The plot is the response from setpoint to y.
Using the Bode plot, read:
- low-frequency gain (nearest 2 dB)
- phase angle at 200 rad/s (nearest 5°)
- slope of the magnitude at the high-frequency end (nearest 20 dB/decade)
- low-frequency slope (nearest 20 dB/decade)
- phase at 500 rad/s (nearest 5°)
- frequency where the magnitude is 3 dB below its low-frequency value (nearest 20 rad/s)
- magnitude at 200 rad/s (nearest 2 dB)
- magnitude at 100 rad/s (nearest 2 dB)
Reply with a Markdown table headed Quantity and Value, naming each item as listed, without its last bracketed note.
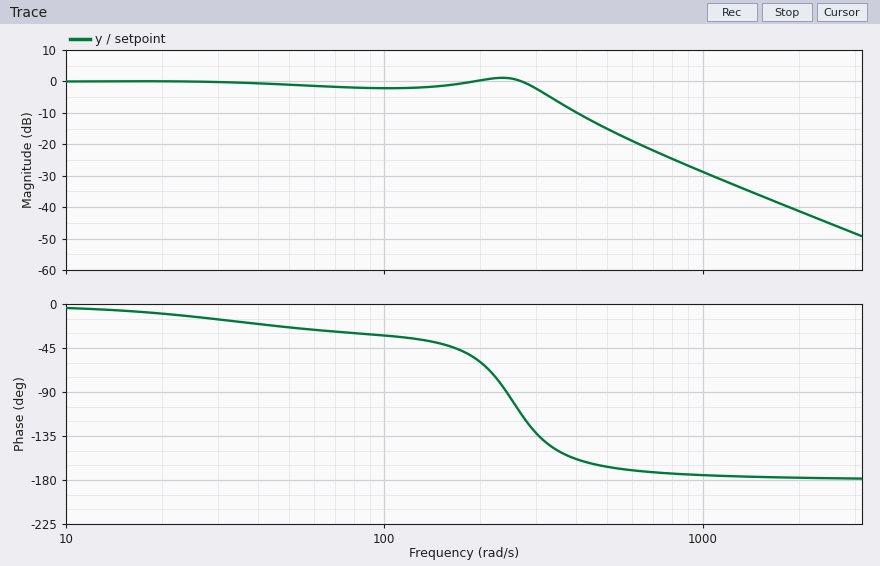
| Quantity | Value |
|---|---|
| low-frequency gain | 0 dB |
| phase angle at 200 rad/s | -60° |
| slope of the magnitude at the high-frequency end | -40 dB/decade |
| low-frequency slope | 0 dB/decade |
| phase at 500 rad/s | -165° |
| frequency where the magnitude is 3 dB below its low-frequency value | 300 rad/s |
| magnitude at 200 rad/s | 0 dB |
| magnitude at 100 rad/s | -2 dB |
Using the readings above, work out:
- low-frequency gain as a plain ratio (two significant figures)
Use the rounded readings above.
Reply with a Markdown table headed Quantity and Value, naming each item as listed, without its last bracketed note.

| Quantity | Value |
|---|---|
| low-frequency gain as a plain ratio | 1.0 |
